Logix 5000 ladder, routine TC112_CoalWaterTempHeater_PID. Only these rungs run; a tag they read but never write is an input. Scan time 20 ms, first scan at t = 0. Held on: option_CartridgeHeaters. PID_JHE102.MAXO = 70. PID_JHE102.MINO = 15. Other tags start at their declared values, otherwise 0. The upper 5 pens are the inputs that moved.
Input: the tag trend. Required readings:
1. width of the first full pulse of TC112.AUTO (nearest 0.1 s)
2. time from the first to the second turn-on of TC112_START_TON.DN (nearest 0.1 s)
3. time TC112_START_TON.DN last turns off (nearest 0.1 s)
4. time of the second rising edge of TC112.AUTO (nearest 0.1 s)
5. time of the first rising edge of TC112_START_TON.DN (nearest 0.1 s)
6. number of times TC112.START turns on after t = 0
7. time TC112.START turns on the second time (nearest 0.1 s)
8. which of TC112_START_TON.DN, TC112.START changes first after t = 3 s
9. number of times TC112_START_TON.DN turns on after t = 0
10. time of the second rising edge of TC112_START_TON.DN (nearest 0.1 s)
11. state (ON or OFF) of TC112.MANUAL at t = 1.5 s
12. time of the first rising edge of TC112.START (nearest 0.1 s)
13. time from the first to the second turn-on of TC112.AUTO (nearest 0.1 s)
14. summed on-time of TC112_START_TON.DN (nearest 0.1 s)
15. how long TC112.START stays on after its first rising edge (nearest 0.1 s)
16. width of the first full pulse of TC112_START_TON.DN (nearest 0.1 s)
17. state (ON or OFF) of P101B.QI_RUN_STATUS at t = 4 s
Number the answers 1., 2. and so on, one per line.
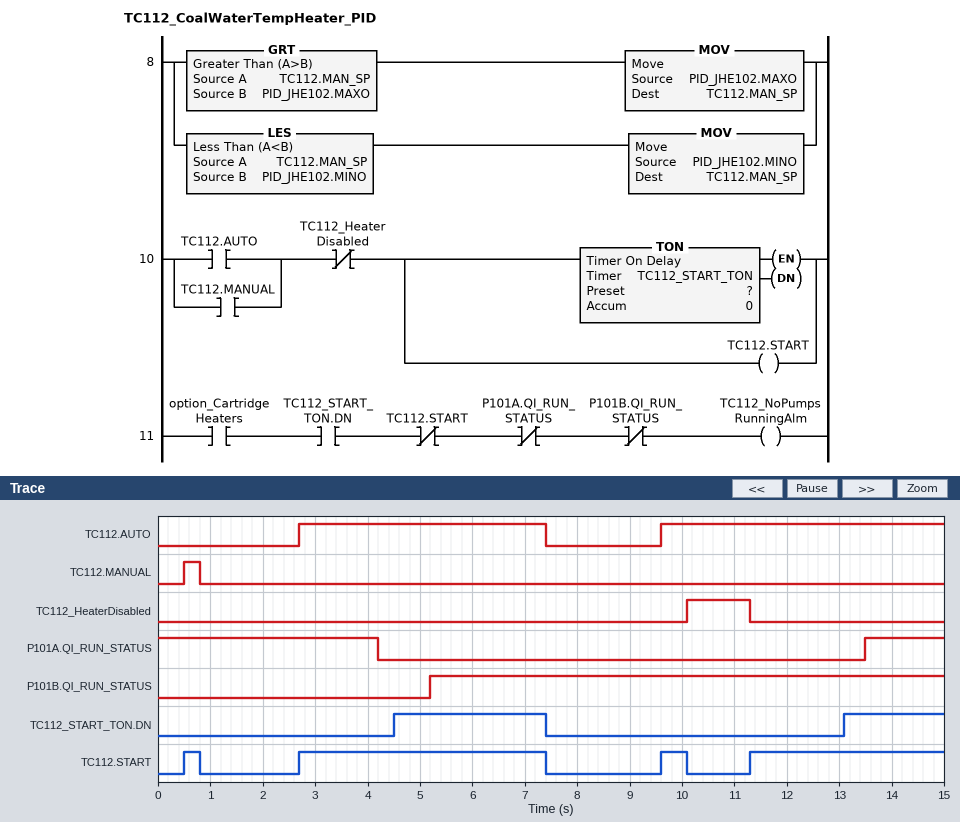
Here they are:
1. 4.7 s
2. 8.6 s
3. 7.4 s
4. 9.6 s
5. 4.5 s
6. 4
7. 2.7 s
8. TC112_START_TON.DN
9. 2
10. 13.1 s
11. OFF
12. 0.5 s
13. 6.9 s
14. 4.8 s
15. 0.3 s
16. 2.9 s
17. OFF
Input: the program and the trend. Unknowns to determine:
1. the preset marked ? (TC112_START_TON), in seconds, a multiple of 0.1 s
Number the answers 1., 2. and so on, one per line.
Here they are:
1. 1.8 s
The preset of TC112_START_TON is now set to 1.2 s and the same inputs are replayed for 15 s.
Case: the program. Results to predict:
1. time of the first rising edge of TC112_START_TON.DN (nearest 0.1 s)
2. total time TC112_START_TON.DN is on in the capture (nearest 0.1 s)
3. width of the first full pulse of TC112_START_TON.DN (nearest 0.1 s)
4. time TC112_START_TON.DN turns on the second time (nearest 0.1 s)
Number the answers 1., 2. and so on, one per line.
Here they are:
1. 3.9 s
2. 6.0 s
3. 3.5 s
4. 12.5 s
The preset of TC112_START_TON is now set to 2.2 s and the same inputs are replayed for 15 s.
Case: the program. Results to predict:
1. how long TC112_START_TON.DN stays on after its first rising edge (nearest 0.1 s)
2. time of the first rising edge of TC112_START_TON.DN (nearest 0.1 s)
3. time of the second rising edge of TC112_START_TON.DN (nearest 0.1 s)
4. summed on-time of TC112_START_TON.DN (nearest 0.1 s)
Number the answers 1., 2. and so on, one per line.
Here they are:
1. 2.5 s
2. 4.9 s
3. 13.5 s
4. 4.0 s
